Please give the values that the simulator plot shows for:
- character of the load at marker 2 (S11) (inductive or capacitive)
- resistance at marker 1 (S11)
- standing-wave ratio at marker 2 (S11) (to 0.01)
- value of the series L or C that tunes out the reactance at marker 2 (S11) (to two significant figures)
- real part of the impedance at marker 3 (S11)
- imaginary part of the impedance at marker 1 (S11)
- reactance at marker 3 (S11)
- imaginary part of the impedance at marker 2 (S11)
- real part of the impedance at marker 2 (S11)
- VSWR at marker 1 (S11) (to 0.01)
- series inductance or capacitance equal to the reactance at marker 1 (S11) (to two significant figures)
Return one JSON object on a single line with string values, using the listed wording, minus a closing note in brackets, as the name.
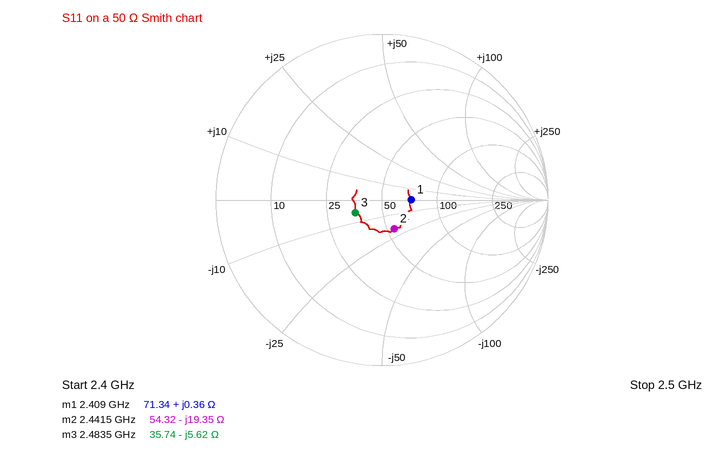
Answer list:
{"character of the load at marker 2 (S11)": "capacitive", "resistance at marker 1": "71.34 Ω", "standing-wave ratio at marker 2 (S11)": "1.46", "value of the series L or C that tunes out the reactance at marker 2 (S11)": "1.3 nH", "real part of the impedance at marker 3": "35.74 Ω", "imaginary part of the impedance at marker 1": "+0.36 Ω", "reactance at marker 3": "-5.62 Ω", "imaginary part of the impedance at marker 2": "-19.35 Ω", "real part of the impedance at marker 2": "54.32 Ω", "VSWR at marker 1 (S11)": "1.43", "series inductance or capacitance equal to the reactance at marker 1 (S11)": "24 pH"}
